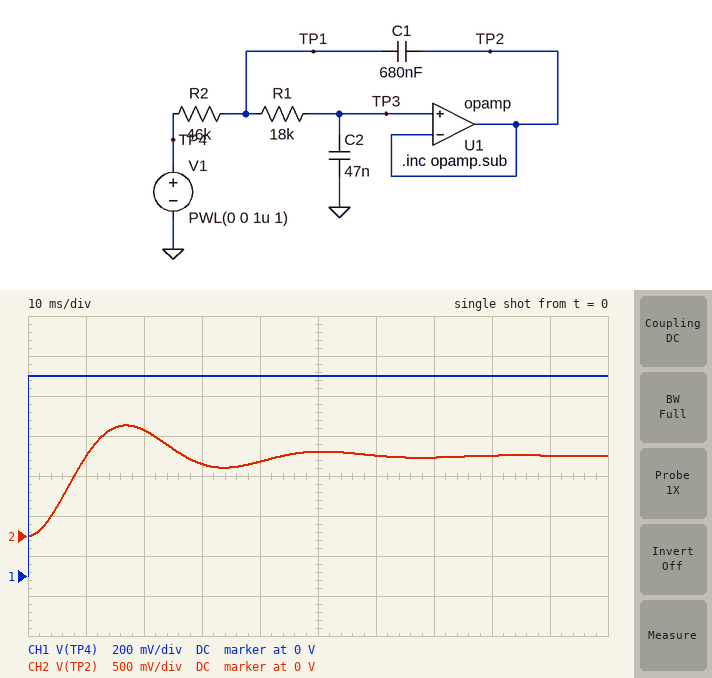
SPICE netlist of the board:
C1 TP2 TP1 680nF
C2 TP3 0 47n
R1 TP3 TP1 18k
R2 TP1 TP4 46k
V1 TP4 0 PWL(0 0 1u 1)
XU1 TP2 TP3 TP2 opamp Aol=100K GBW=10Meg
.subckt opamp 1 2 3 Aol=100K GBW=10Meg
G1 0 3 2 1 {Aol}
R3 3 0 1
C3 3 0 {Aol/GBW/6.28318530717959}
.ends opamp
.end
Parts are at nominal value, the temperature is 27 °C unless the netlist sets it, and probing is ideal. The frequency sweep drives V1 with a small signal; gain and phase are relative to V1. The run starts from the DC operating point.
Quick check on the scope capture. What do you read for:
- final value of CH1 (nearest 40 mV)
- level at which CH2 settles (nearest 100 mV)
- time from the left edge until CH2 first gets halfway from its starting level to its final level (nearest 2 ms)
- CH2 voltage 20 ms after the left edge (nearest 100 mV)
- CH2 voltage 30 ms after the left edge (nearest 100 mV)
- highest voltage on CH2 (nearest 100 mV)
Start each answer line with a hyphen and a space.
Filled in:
- 1.00 V
- 1.0 V
- 6 ms
- 1.3 V
- 900 mV
- 1.4 V
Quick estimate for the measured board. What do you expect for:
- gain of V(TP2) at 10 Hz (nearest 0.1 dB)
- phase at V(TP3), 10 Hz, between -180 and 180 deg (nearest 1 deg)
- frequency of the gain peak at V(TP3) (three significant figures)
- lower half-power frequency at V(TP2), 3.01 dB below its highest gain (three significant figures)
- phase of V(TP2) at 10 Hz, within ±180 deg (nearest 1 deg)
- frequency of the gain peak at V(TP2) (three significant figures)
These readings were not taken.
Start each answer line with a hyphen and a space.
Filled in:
- 0.8 dB
- -12 deg
- 28.2 Hz
- 16.1 Hz
- -12 deg
- 28.2 Hz
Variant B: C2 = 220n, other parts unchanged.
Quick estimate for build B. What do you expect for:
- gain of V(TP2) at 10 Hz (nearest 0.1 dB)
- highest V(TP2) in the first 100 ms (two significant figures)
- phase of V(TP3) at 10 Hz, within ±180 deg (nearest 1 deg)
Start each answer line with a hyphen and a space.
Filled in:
- -0.2 dB
- 1.1 V
- -60 deg
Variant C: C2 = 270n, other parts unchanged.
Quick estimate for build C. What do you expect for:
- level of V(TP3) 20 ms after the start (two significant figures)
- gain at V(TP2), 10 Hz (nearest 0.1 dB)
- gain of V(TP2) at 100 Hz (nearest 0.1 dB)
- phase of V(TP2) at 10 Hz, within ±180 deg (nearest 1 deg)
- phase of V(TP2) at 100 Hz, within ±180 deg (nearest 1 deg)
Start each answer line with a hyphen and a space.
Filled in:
- 580 mV
- -1.3 dB
- -35.6 dB
- -70 deg
- -170 deg
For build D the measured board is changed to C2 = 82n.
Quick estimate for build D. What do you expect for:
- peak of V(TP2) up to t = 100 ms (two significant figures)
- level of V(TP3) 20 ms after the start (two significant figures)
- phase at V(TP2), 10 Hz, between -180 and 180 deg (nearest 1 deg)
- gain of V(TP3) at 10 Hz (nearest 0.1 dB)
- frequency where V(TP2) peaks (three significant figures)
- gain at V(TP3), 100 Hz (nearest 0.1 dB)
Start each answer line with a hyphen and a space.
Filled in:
- 1.3 V
- 1.2 V
- -22 deg
- 1.1 dB
- 19.6 Hz
- -24.9 dB
